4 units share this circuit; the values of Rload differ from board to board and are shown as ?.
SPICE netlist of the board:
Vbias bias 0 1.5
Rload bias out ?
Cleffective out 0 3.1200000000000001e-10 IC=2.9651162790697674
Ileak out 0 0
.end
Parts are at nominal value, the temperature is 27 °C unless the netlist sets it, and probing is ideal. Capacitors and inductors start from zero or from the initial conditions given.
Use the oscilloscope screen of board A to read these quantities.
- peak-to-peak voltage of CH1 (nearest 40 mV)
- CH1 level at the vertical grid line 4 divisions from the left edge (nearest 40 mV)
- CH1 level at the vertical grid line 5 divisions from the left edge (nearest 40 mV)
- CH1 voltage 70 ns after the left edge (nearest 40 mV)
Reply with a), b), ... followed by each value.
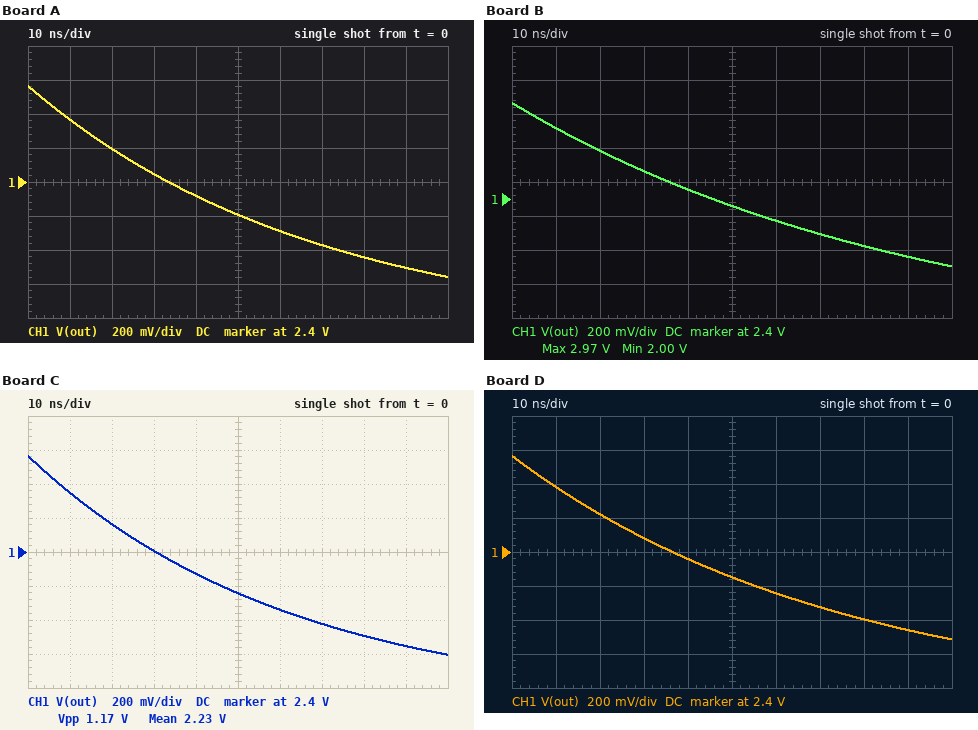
a) 1.12 V
b) 2.32 V
c) 2.20 V
d) 2.04 V
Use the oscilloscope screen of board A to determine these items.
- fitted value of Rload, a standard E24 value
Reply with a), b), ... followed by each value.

a) 220 Ω
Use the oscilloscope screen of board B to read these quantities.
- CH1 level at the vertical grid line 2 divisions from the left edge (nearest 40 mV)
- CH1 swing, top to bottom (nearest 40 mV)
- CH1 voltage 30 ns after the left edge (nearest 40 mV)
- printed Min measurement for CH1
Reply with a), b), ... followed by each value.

a) 2.68 V
b) 960 mV
c) 2.56 V
d) 2.00 V
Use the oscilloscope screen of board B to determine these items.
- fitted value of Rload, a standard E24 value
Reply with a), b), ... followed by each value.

a) 300 Ω
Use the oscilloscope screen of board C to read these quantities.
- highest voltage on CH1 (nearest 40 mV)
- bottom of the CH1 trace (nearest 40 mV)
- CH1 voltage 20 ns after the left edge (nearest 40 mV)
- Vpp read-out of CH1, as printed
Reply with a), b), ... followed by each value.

a) 2.96 V
b) 1.80 V
c) 2.56 V
d) 1.17 V
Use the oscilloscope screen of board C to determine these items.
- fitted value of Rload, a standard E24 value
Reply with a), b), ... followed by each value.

a) 200 Ω
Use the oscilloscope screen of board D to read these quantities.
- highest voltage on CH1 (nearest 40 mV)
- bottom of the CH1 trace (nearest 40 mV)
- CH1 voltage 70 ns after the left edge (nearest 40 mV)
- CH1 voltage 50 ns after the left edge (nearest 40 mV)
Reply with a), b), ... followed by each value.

a) 2.96 V
b) 1.88 V
c) 2.08 V
d) 2.24 V
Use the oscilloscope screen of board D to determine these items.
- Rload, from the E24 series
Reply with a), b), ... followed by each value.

a) 240 Ω
